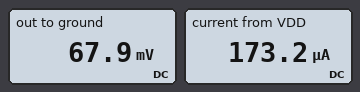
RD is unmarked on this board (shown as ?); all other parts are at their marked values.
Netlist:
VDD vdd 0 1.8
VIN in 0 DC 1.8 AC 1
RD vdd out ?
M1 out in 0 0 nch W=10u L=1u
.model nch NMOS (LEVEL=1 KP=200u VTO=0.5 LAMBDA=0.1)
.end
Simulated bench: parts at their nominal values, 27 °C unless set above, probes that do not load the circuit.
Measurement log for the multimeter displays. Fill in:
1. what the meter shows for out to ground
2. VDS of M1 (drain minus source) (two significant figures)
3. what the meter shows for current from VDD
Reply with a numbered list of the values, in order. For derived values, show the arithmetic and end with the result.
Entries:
1. 67.9 mV
2. 67.9 mV = 68 mV
3. 173.2 µA
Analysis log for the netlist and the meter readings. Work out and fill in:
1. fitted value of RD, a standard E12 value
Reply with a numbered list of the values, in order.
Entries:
1. 10 kΩ
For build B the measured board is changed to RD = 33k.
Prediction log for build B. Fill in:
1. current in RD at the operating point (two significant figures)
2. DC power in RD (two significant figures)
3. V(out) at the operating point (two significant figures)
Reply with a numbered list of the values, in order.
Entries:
1. 54 µA
2. 96 µW
3. 21 mV
